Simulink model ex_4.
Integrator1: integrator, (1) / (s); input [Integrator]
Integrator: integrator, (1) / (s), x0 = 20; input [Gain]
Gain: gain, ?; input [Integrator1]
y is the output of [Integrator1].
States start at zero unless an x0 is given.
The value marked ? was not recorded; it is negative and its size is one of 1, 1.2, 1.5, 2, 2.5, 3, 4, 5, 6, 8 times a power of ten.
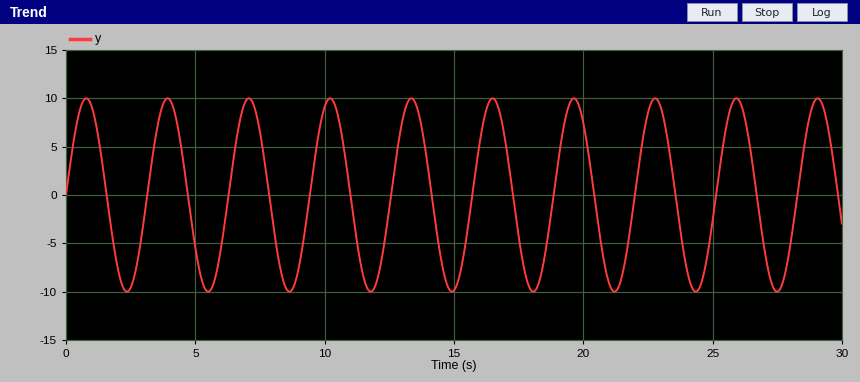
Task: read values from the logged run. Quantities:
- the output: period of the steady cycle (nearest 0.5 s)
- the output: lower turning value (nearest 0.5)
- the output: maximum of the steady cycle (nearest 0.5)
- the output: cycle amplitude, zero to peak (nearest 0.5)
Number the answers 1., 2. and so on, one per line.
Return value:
1. 3.0 s
2. -10.0
3. 10.0
4. 10.0
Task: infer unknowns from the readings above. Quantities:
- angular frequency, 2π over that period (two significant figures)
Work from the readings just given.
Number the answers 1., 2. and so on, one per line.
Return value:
1. 2.1 rad/s
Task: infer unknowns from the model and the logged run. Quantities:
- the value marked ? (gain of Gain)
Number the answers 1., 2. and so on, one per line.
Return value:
1. -4
